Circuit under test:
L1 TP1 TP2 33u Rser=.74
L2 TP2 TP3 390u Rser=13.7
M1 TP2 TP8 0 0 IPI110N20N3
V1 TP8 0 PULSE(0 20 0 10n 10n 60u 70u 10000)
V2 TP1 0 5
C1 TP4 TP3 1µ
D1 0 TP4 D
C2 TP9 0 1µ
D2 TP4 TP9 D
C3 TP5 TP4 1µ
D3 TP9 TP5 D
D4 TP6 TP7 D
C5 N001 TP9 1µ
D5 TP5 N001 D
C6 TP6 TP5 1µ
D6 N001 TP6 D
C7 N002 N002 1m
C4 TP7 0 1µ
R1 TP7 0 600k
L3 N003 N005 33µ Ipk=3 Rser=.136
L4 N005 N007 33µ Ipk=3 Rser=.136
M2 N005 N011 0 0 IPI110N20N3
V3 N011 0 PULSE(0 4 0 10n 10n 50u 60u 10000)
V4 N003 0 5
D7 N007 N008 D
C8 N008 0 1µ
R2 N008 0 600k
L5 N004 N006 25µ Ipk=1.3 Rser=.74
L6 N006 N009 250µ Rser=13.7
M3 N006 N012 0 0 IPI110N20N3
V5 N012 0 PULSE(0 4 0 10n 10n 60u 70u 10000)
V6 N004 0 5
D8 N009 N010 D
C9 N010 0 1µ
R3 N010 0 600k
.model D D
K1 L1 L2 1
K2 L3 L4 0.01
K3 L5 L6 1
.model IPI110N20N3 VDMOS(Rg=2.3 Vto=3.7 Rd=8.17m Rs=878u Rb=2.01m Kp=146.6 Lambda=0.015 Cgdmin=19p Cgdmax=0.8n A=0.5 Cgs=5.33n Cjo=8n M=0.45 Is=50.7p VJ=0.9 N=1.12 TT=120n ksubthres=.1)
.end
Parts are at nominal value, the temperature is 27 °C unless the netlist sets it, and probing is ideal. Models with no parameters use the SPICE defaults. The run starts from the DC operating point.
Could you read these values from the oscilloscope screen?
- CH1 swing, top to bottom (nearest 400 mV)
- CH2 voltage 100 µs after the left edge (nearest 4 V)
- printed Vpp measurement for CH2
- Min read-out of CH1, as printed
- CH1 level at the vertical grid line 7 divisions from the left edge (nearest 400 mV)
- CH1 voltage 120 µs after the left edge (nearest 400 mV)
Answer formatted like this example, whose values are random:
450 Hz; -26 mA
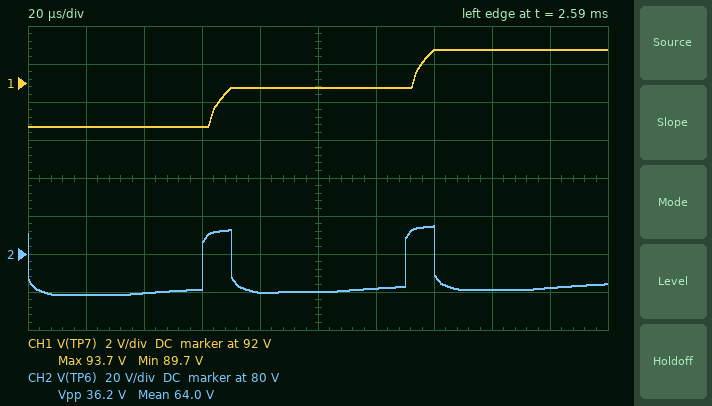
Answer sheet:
4.0 V; 60 V; 36.2 V; 89.7 V; 93.6 V; 91.6 V
